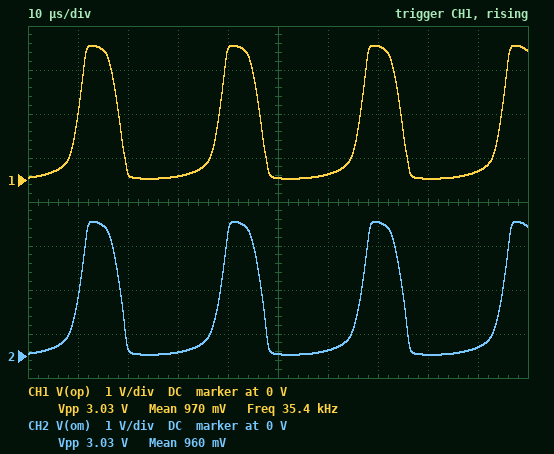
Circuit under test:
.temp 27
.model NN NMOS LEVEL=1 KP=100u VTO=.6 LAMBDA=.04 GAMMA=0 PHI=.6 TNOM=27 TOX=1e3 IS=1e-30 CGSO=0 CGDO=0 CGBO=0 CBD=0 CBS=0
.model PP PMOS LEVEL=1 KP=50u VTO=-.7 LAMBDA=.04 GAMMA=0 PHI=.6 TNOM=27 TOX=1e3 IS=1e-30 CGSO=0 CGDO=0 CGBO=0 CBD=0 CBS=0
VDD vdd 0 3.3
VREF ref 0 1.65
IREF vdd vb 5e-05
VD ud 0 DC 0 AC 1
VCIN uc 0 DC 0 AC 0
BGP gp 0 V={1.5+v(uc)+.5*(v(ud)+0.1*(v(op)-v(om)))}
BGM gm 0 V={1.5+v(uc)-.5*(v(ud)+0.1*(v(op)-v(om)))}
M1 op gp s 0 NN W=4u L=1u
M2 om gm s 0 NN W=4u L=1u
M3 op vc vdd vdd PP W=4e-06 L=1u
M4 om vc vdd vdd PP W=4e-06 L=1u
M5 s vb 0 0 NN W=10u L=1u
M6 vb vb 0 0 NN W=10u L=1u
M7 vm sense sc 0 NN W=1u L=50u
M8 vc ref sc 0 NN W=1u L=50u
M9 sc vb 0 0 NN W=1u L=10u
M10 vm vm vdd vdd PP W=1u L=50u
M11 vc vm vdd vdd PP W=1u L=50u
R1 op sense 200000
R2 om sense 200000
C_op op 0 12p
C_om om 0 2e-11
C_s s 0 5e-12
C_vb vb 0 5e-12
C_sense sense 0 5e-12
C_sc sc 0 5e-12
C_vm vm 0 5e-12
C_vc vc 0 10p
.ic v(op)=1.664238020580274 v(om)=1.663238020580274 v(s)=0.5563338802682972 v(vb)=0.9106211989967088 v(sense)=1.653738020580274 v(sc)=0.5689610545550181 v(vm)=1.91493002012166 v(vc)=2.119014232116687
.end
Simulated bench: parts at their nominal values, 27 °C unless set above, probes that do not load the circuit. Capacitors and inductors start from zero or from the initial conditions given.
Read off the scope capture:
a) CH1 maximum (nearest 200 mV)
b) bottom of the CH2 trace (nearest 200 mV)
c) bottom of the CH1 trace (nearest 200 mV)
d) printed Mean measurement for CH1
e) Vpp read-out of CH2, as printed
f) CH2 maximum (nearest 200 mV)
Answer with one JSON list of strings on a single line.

["3.0 V", "0 V", "0 V", "970 mV", "3.03 V", "3.0 V"]
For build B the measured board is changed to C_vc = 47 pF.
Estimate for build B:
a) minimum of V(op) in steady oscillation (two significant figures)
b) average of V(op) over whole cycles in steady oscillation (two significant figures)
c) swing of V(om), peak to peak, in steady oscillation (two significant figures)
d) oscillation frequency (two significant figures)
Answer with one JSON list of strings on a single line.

["210 mV", "1.3 V", "2.7 V", "26 kHz"]
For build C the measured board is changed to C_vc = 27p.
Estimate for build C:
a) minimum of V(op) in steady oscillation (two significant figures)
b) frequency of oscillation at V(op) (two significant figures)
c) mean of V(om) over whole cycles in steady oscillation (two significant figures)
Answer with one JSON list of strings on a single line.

["150 mV", "29 kHz", "1.2 V"]
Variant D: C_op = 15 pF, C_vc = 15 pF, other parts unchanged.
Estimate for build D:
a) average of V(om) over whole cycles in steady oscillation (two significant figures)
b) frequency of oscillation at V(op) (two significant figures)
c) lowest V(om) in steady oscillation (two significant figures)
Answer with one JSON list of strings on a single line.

["1.0 V", "32 kHz", "73 mV"]
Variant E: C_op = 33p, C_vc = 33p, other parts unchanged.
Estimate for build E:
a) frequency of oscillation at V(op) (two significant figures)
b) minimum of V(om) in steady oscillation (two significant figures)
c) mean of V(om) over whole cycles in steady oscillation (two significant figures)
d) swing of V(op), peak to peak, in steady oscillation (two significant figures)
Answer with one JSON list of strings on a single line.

["25 kHz", "160 mV", "1.3 V", "2.8 V"]
